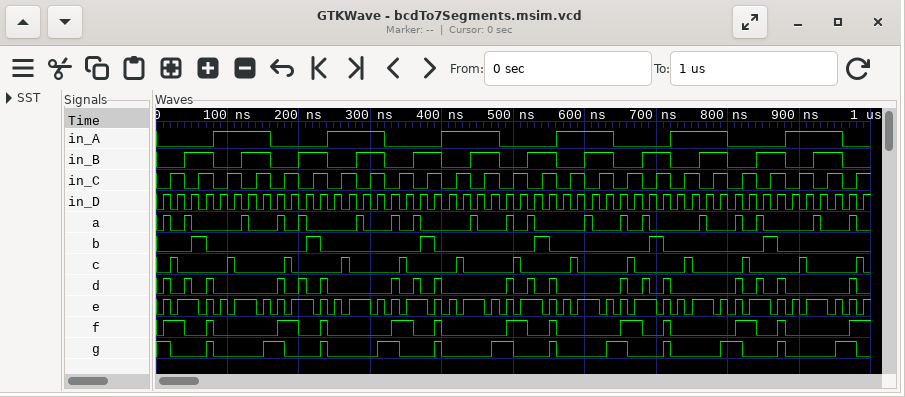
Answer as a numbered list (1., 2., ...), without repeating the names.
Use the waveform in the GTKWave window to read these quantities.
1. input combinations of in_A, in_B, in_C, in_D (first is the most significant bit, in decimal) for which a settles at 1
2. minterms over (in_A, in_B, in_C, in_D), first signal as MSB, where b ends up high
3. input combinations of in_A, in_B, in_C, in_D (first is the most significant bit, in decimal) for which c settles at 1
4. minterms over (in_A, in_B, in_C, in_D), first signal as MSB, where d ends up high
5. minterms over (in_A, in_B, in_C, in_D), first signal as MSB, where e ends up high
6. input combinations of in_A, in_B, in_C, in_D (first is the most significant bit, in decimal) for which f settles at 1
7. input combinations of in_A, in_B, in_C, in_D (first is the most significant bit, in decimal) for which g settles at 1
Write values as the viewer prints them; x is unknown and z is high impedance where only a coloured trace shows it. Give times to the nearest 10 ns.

1. 1, 4, 12
2. 5, 6
3. 2, 10
4. 1, 4, 7
5. 1, 3, 4, 5, 7, 9, 11, 12, 13, 15
6. 1, 2, 3, 7
7. 0, 1, 7, 15
